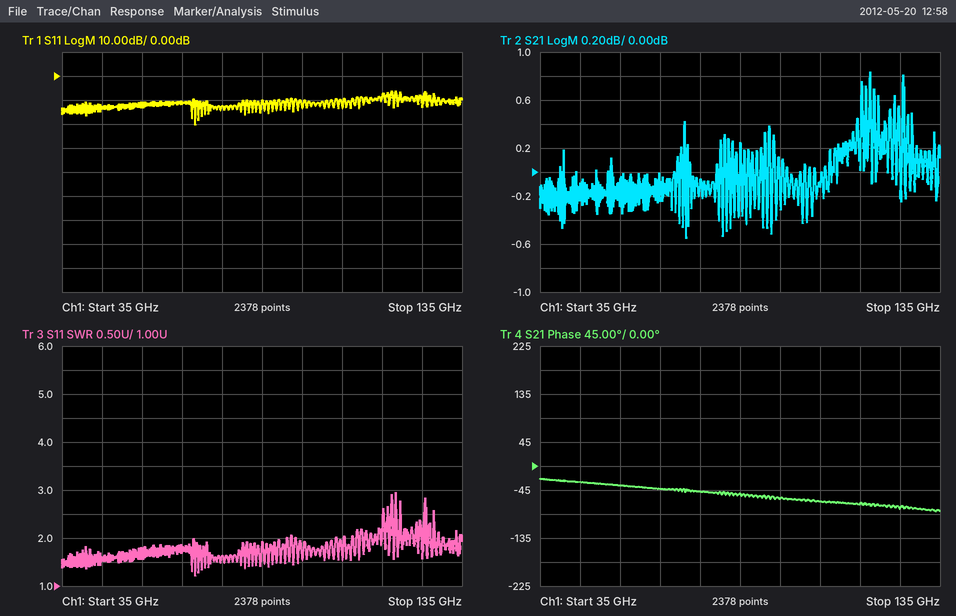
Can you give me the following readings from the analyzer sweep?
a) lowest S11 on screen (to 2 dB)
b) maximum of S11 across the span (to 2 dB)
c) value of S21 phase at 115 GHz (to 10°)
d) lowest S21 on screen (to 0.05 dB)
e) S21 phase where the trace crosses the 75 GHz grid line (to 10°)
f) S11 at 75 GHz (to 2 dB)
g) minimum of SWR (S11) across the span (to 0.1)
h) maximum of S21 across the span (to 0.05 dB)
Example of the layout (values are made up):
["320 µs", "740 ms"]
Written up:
["-20 dB", "-6 dB", "-70°", "-0.55 dB", "-50°", "-12 dB", "1.2", "0.85 dB"]
